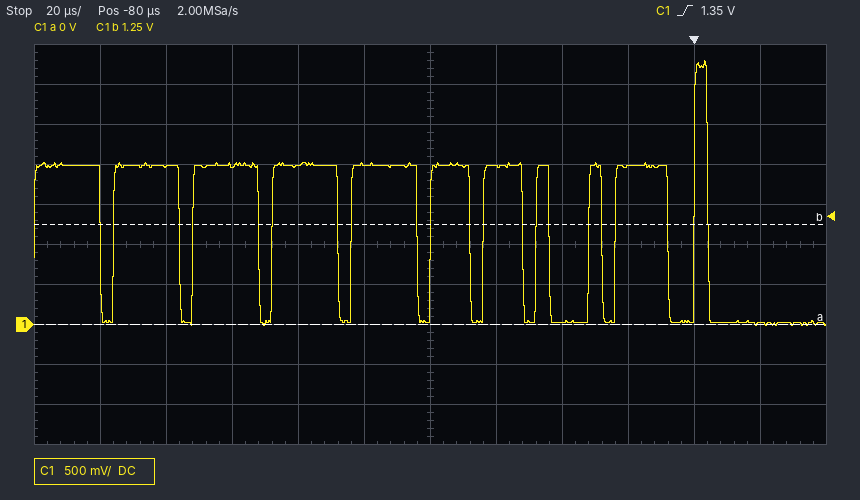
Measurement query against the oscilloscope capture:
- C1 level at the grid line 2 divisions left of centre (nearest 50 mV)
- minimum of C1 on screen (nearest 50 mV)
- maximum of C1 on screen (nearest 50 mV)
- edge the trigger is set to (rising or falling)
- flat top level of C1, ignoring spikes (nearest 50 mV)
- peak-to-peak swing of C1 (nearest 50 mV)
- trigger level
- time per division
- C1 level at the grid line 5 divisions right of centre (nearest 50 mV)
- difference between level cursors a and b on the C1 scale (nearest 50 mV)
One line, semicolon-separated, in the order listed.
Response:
2.00 V; 0 mV; 3.30 V; rising; 2.00 V; 3.30 V; 1.35 V; 20 µs; 0 mV; 1.25 V
